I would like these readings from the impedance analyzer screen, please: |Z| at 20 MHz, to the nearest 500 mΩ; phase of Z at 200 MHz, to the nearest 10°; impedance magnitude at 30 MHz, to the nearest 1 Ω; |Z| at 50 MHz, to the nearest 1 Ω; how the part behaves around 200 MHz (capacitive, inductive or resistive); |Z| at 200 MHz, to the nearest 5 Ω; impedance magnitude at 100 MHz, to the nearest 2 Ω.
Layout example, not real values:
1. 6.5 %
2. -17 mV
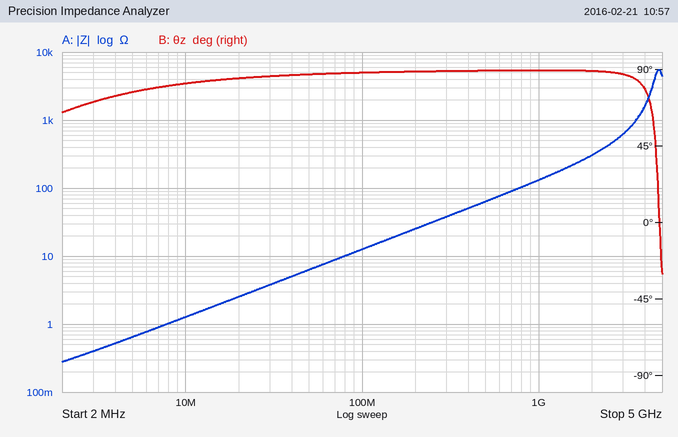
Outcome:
1. 2.5 Ω
2. 90°
3. 4 Ω
4. 6 Ω
5. inductive
6. 25 Ω
7. 12 Ω
